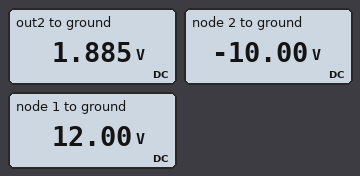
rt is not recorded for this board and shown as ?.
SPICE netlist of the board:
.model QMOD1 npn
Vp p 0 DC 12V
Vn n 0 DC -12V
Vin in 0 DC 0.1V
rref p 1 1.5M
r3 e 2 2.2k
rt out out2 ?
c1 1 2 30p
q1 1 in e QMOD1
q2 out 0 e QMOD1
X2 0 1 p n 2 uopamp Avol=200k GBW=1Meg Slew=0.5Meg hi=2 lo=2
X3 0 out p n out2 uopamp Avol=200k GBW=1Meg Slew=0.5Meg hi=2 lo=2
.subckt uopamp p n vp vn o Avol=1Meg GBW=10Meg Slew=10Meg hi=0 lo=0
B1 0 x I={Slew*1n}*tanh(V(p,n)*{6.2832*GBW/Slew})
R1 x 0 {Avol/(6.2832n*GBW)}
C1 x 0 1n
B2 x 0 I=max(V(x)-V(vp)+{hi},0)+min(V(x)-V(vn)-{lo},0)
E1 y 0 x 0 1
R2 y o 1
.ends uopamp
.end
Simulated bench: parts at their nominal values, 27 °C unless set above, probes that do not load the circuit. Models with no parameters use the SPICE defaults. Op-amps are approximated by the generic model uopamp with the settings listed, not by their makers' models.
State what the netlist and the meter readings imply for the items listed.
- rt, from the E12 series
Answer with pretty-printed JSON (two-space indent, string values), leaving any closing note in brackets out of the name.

{
  "rt, from the E12 series": "22 kΩ"
}
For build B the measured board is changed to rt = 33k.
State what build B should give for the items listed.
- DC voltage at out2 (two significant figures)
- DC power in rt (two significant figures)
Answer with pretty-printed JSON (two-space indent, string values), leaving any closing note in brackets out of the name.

{
  "DC voltage at out2": "2.8 V",
  "DC power in rt": "240 µW"
}
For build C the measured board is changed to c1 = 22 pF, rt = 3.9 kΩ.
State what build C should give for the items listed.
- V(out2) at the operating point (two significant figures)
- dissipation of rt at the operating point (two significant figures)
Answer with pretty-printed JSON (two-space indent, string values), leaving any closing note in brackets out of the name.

{
  "V(out2) at the operating point": "330 mV",
  "dissipation of rt at the operating point": "29 µW"
}
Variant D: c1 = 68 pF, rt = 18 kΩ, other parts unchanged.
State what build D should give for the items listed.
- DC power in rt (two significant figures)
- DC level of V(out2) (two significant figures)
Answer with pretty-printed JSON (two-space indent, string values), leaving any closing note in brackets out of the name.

{
  "DC power in rt": "130 µW",
  "DC level of V(out2)": "1.5 V"
}
